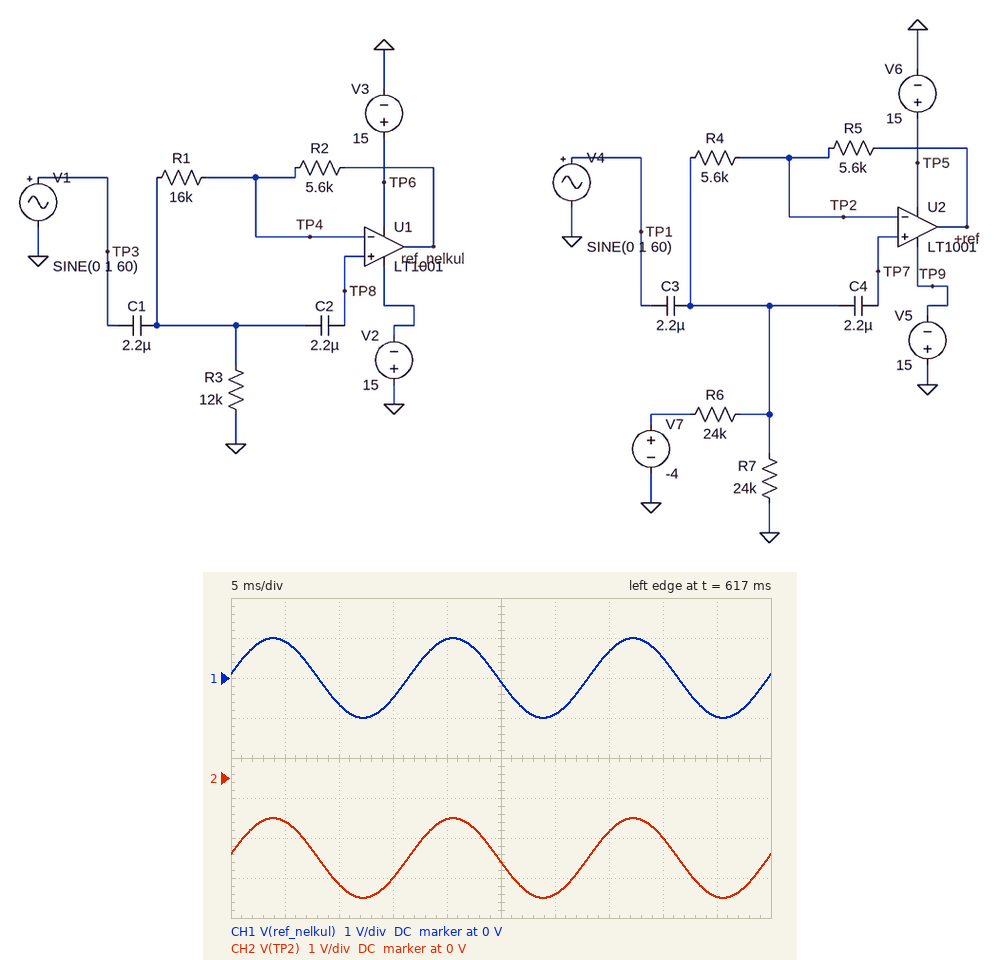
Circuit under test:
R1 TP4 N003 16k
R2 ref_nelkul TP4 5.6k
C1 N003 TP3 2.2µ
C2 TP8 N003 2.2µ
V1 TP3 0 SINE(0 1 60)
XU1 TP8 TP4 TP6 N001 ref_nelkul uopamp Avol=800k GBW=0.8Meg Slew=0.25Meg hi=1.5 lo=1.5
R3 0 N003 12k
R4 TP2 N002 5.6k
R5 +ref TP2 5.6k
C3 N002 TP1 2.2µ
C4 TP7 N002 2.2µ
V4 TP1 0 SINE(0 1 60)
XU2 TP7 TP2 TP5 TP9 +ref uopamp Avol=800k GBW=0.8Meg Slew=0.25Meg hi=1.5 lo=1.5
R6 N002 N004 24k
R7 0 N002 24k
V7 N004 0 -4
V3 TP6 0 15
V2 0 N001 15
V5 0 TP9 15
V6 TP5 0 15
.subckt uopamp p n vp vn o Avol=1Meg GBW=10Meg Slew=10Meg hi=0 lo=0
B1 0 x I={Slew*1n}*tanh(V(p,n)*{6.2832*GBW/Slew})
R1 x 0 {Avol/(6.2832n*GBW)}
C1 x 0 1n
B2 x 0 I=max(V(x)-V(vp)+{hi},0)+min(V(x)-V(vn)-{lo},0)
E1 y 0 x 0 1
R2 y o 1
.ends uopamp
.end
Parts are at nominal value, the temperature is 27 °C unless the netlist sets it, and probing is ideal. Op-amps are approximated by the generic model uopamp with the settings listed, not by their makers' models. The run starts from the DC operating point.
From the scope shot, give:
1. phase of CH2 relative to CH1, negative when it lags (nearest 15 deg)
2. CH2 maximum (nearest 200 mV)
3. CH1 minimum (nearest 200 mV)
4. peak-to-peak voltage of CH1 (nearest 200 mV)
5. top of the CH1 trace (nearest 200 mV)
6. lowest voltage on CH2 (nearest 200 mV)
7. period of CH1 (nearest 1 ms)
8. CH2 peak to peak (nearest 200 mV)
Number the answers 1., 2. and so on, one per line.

1. 0 deg
2. -1.0 V
3. -1.0 V
4. 2.0 V
5. 1.0 V
6. -3.0 V
7. 17 ms
8. 2.0 V
